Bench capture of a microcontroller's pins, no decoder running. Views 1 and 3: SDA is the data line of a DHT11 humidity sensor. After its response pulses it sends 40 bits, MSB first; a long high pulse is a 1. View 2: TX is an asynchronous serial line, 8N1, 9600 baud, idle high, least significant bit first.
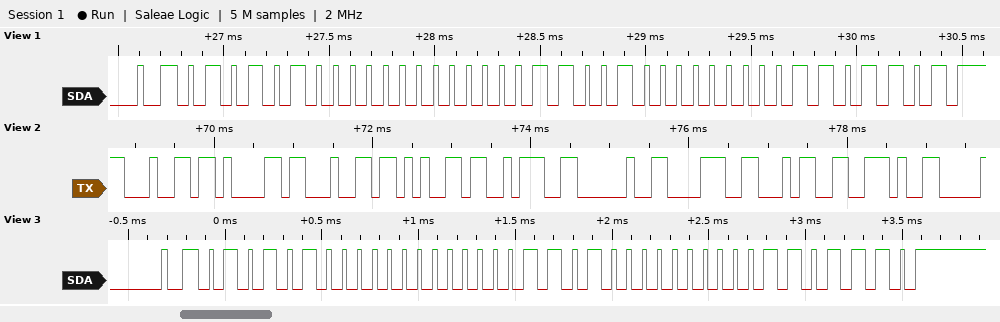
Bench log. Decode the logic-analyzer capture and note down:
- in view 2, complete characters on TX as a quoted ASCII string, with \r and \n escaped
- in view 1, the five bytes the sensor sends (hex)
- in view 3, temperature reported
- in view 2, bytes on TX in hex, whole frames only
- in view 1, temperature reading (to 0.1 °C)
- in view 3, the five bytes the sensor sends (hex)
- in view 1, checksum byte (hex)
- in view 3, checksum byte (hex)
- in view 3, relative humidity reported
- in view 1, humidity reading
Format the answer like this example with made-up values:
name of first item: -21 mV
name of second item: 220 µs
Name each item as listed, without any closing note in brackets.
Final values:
in view 2, complete characters on TX as a quoted ASCII string, with \r and \n escaped: "dade: 84."
in view 1, the five bytes the sensor sends: 54 00 19 00 6D
in view 3, temperature reported: 26.0 °C
in view 2, bytes on TX in hex, whole frames only: 64 61 64 65 3A 20 38 34 2E
in view 1, temperature reading: 25.0 °C
in view 3, the five bytes the sensor sends: 54 00 1A 00 6E
in view 1, checksum byte: 0x6D
in view 3, checksum byte: 0x6E
in view 3, relative humidity reported: 84 %
in view 1, humidity reading: 84 %
